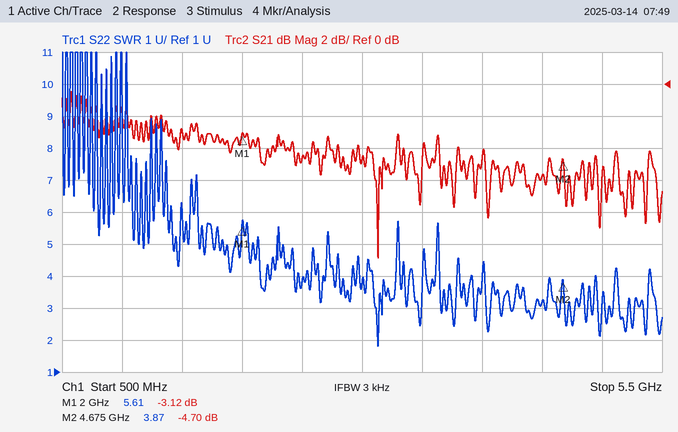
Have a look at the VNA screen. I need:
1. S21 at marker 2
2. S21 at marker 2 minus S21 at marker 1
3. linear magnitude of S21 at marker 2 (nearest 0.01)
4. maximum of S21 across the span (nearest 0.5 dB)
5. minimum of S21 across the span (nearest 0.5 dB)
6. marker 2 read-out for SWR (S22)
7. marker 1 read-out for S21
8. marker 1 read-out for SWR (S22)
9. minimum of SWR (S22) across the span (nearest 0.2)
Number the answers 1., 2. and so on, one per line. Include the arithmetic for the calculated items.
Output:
1. -4.70 dB
2. -4.7 − (-3.12) = -1.58 dB
3. 10^(-4.7/20) ≈ 0.58
4. -0.5 dB
5. -11.0 dB
6. 3.87
7. -3.12 dB
8. 5.61
9. 1.8
